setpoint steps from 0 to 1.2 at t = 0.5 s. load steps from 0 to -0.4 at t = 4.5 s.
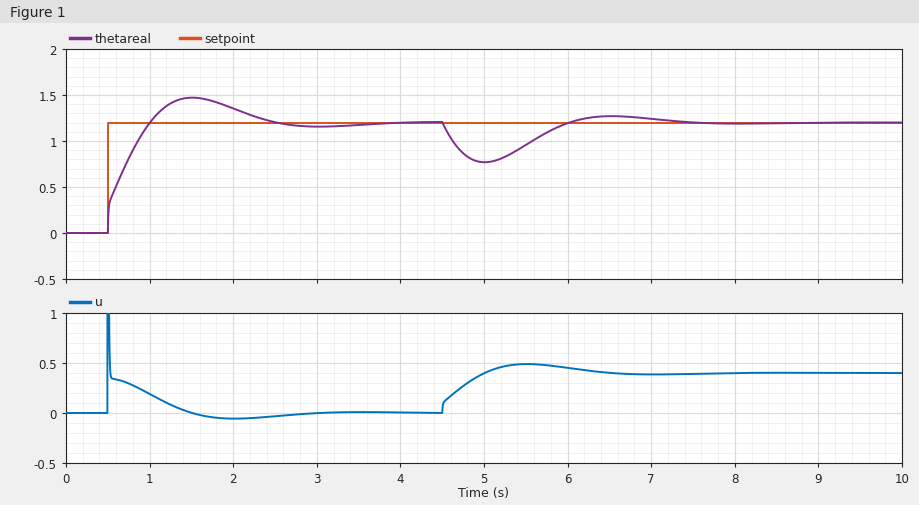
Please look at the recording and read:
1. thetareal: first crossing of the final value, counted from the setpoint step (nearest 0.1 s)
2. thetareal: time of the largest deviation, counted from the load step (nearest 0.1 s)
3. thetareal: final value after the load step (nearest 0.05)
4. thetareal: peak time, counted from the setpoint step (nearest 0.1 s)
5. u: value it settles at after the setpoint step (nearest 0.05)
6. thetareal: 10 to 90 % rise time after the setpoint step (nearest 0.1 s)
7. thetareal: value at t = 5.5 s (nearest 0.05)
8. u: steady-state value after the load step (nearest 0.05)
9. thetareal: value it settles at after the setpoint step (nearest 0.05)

0.5 s
0.5 s
1.20
1.0 s
0.00
0.4 s
0.95
0.40
1.20
